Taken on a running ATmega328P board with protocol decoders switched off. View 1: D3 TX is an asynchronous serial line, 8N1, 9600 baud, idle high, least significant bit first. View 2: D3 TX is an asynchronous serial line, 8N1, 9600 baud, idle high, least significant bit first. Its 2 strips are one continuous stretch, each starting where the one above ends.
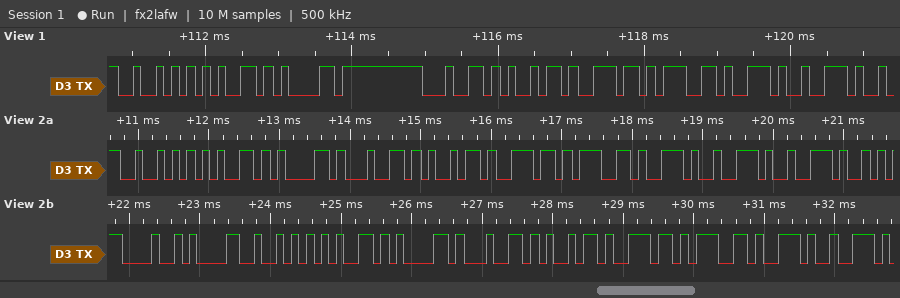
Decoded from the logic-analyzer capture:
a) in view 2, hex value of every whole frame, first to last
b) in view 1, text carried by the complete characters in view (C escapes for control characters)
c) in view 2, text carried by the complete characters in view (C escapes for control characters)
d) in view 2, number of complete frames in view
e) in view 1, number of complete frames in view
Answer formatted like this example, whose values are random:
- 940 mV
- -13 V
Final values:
- 52 65 61 64 69 6E 67 2E 2E 2E 0D 0A 52 65 61 64 69 6E 67 2E
- "Reading.."
- "Reading...\r\nReading."
- 20
- 9
